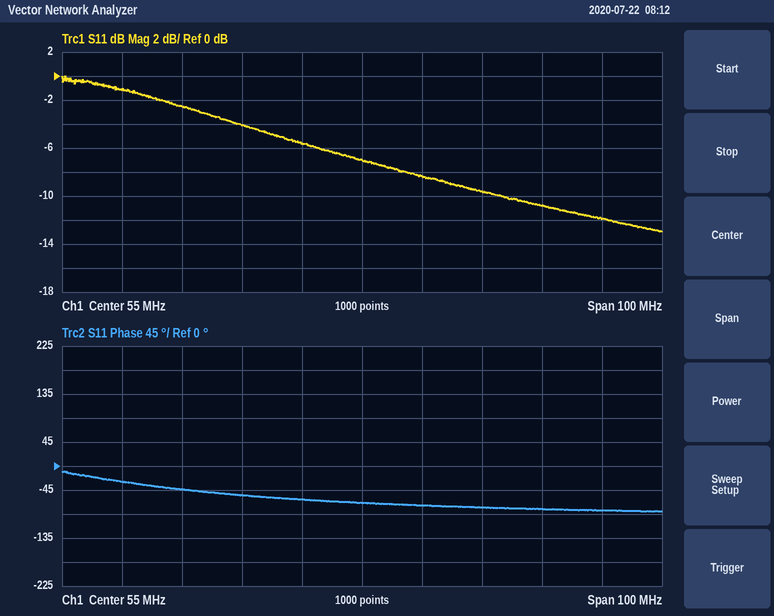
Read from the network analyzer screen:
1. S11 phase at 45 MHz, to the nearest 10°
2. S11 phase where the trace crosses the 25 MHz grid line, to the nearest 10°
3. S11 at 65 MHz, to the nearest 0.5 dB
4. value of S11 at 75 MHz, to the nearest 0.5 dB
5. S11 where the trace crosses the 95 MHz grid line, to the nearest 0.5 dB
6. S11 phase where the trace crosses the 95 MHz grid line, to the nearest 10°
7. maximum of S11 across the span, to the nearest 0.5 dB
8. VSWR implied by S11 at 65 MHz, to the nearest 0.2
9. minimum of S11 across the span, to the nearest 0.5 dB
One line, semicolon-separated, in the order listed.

-60°; -40°; -8.5 dB; -9.5 dB; -12.0 dB; -80°; 0.0 dB; 2.2; -13.0 dB
